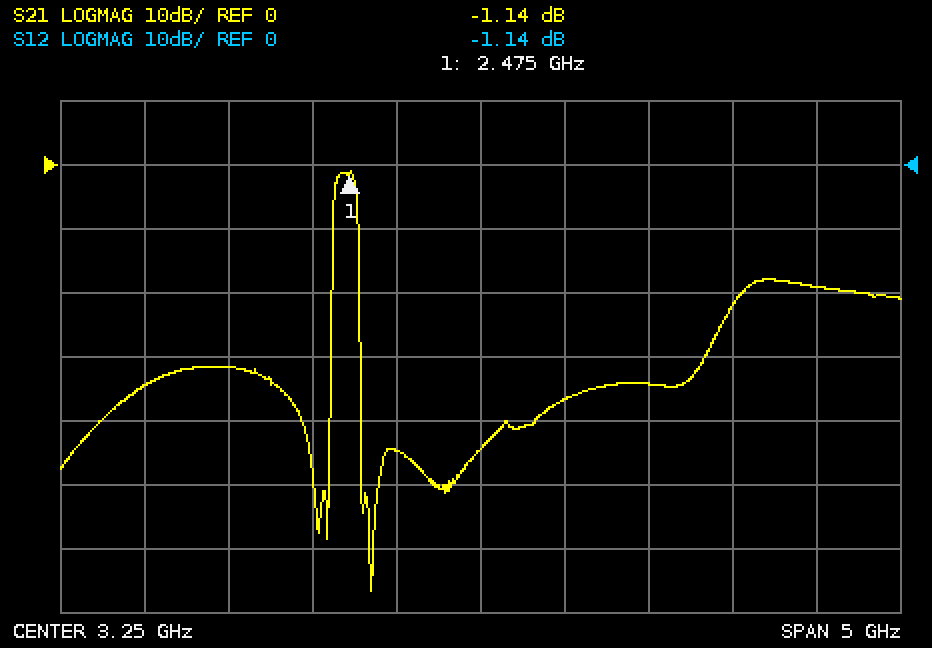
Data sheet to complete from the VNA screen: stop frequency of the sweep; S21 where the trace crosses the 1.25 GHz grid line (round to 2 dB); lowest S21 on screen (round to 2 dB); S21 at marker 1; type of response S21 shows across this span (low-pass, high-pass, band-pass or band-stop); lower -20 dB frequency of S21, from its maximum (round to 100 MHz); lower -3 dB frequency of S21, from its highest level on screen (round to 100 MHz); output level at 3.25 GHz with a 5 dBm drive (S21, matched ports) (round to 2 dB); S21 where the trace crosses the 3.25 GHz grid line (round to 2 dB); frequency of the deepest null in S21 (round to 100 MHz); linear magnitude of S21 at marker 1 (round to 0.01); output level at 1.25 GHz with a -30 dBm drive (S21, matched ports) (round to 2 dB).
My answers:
5.75 GHz
-34 dB
-66 dB
-1.14 dB
band-pass
2.4 GHz
2.4 GHz
-40 dBm
-44 dB
2.6 GHz
0.88
-64 dBm
